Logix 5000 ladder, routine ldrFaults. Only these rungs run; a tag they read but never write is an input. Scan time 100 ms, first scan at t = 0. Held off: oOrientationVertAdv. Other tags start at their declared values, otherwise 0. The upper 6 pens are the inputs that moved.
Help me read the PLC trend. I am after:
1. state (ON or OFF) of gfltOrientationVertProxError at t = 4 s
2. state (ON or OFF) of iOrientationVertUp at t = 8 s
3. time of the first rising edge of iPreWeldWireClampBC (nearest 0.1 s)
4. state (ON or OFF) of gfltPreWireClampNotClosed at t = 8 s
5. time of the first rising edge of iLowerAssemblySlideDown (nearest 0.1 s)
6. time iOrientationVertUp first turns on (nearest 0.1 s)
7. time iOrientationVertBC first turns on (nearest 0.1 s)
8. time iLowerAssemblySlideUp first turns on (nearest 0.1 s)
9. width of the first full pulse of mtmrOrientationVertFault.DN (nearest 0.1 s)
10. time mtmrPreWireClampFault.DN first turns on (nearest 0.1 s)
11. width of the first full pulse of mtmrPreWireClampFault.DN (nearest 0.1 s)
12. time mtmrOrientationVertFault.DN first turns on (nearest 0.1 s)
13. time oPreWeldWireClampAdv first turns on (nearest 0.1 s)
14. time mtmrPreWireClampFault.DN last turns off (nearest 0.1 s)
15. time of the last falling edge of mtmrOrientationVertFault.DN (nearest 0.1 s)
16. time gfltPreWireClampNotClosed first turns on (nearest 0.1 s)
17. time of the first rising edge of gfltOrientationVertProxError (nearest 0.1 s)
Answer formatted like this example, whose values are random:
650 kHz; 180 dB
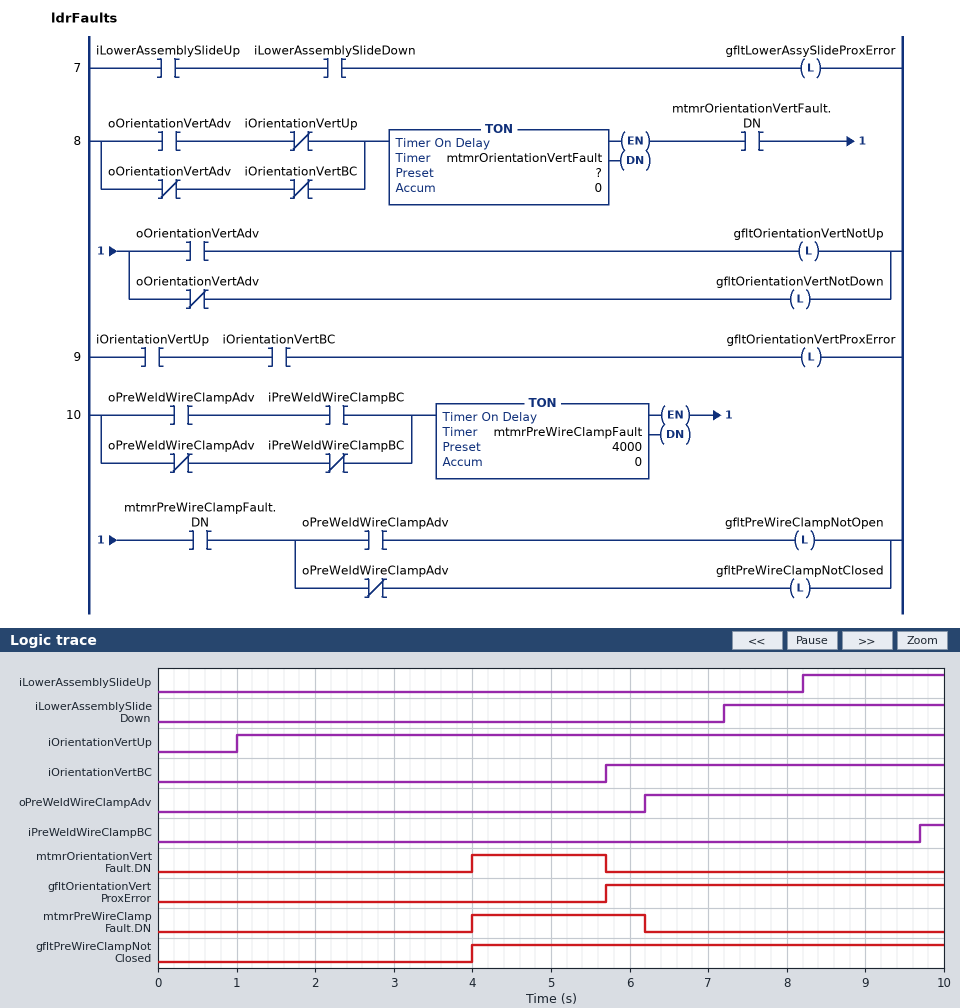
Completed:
OFF; ON; 9.7 s; ON; 7.2 s; 1.0 s; 5.7 s; 8.2 s; 1.7 s; 4.0 s; 2.2 s; 4.0 s; 6.2 s; 6.2 s; 5.7 s; 4.0 s; 5.7 s
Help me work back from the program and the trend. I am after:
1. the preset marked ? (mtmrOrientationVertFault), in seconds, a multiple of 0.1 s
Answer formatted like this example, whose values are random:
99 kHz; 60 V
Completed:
4.0 s
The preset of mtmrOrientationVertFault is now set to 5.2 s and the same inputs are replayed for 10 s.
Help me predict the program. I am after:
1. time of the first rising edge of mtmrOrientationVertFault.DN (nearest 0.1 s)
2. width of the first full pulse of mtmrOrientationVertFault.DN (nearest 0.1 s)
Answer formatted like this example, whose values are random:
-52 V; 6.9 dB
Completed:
5.2 s; 0.5 s
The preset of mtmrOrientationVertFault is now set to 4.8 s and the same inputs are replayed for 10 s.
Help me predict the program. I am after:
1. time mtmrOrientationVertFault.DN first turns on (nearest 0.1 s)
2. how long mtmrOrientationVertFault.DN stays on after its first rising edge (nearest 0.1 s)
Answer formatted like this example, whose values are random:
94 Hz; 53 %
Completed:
4.8 s; 0.9 s
